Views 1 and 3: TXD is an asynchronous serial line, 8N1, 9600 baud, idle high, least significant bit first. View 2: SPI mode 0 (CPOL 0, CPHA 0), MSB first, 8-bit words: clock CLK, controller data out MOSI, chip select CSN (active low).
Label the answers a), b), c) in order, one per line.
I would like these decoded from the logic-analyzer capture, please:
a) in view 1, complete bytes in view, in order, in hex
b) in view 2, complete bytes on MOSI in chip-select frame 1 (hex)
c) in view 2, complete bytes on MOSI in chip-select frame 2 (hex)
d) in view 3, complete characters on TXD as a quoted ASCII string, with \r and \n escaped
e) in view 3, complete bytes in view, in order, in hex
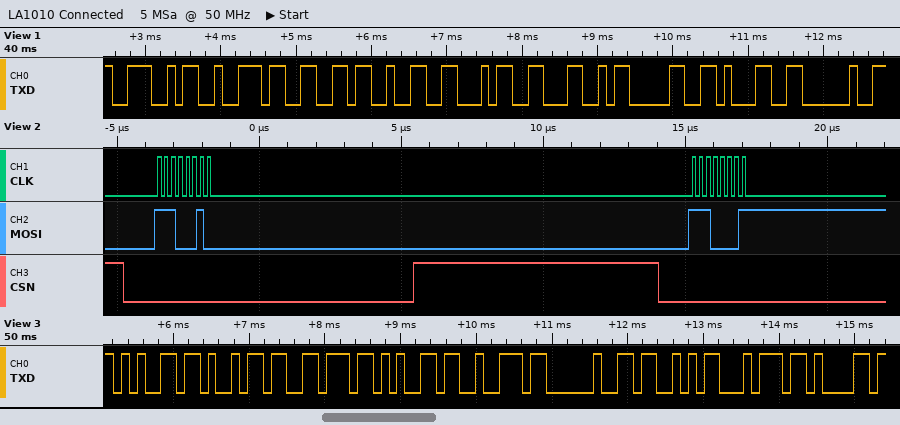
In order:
a) 0x4E 0x72 0x66 0x32 0x34 0x4C 0x30 0x31 0x20
b) 0xE2
c) 0xE1
d) "eiver Sta"
e) 65 69 76 65 72 20 53 74 61
